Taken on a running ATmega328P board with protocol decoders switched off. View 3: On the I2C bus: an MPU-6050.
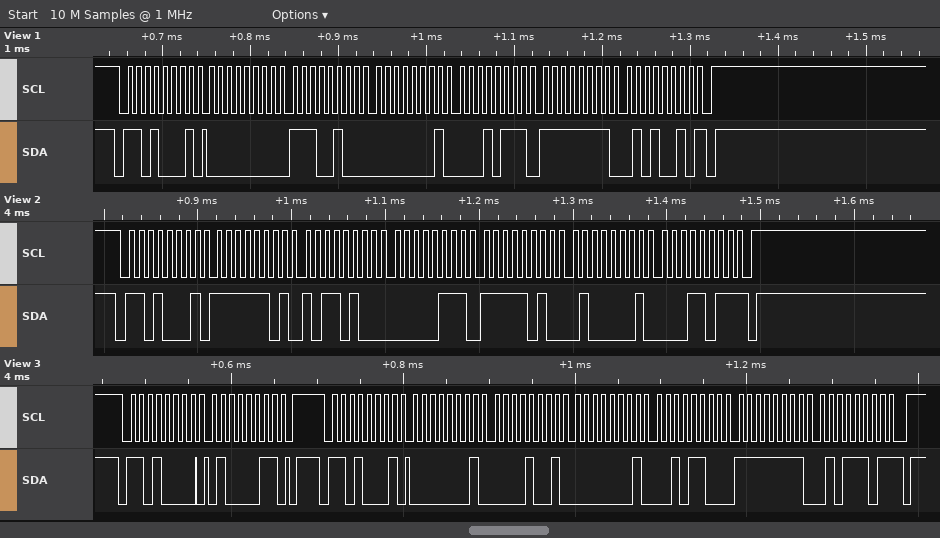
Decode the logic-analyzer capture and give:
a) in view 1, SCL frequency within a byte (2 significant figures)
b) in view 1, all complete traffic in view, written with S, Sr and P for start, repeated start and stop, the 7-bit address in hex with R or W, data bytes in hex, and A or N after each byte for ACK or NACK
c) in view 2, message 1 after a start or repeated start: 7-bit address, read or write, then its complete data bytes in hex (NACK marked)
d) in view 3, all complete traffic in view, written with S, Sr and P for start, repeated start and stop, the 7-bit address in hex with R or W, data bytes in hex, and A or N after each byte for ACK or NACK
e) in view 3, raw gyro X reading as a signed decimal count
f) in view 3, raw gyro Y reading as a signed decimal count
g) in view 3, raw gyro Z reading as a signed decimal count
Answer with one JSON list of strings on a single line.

["100 kHz", "S 68R A 00 A E4 A 01 A 17 A FF A 52 N P", "0x68 read: FD B4 07 FA 41 1B NACK", "S 68W A 43 A P S 68R A 01 A 09 A 01 A 2C A FF A 5D N P", "265", "300", "-163"]
